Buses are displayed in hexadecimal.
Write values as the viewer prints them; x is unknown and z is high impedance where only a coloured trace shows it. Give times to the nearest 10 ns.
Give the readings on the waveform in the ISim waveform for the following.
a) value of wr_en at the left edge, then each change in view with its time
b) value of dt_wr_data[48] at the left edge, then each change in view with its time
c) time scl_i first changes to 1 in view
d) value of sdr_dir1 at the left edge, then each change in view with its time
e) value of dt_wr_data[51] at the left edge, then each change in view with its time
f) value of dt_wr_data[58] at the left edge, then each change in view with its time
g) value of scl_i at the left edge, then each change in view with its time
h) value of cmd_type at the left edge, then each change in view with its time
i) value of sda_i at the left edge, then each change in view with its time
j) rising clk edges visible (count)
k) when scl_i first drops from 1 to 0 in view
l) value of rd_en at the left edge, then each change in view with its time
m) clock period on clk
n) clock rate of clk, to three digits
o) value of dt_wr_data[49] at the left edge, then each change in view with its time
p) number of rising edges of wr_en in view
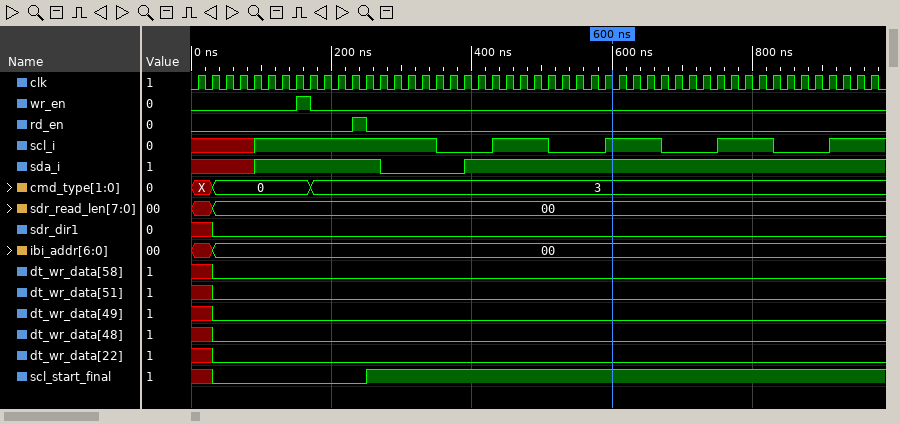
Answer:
0, 1 at 150 ns, 0 at 170 ns
x, 0 at 30 ns
90 ns
x, 0 at 30 ns
x, 0 at 30 ns
x, 0 at 30 ns
x, 1 at 90 ns, 0 at 350 ns, 1 at 430 ns, 0 at 510 ns, 1 at 590 ns, 0 at 670 ns, 1 at 750 ns, 0 at 830 ns, 1 at 910 ns
X, 0 at 30 ns, 3 at 170 ns
x, 1 at 90 ns, 0 at 270 ns, 1 at 390 ns
49
350 ns
0, 1 at 230 ns, 0 at 250 ns
20 ns
50.0 MHz
x, 0 at 30 ns
1
